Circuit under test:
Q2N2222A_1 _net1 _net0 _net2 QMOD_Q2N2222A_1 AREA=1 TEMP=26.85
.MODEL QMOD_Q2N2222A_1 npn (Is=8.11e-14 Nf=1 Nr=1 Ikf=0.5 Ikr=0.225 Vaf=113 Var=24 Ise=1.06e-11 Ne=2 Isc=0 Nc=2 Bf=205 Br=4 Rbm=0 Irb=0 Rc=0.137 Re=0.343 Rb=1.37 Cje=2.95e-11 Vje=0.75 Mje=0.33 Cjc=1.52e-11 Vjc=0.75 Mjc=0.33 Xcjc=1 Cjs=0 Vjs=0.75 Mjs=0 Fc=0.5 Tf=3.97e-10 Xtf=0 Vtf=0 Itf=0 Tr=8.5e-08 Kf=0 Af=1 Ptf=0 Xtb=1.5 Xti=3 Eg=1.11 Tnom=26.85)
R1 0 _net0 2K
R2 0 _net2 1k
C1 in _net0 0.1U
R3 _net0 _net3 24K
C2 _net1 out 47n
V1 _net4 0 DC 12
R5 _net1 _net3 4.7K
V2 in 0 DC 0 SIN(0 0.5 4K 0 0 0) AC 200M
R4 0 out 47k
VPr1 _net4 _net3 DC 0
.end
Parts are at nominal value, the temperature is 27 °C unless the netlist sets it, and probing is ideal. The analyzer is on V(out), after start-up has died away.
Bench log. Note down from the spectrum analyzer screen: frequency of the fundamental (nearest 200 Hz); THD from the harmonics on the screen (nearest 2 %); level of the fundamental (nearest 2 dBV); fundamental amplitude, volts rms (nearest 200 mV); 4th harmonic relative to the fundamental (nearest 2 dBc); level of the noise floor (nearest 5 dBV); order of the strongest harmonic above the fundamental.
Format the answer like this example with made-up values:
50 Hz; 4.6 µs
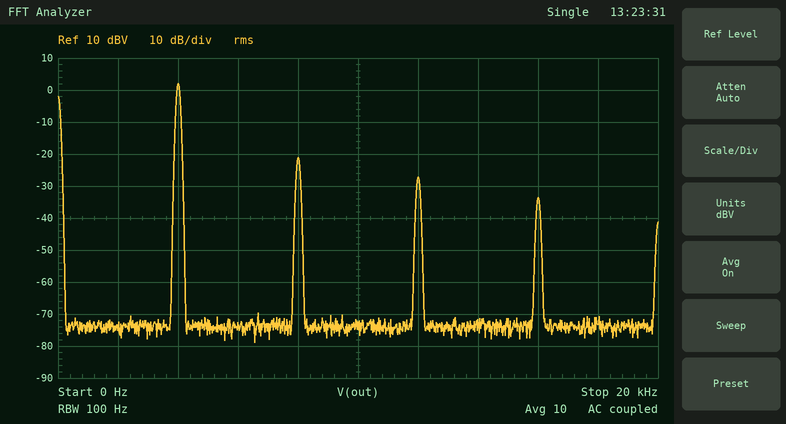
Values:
4.0 kHz; 8 %; 2 dBV; 1.2 V; -36 dBc; -75 dBV; 2
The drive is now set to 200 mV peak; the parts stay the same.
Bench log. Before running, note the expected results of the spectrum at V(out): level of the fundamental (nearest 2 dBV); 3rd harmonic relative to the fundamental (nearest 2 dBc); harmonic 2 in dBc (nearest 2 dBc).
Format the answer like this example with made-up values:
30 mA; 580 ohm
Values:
-6 dBV; -56 dBc; -40 dBc
